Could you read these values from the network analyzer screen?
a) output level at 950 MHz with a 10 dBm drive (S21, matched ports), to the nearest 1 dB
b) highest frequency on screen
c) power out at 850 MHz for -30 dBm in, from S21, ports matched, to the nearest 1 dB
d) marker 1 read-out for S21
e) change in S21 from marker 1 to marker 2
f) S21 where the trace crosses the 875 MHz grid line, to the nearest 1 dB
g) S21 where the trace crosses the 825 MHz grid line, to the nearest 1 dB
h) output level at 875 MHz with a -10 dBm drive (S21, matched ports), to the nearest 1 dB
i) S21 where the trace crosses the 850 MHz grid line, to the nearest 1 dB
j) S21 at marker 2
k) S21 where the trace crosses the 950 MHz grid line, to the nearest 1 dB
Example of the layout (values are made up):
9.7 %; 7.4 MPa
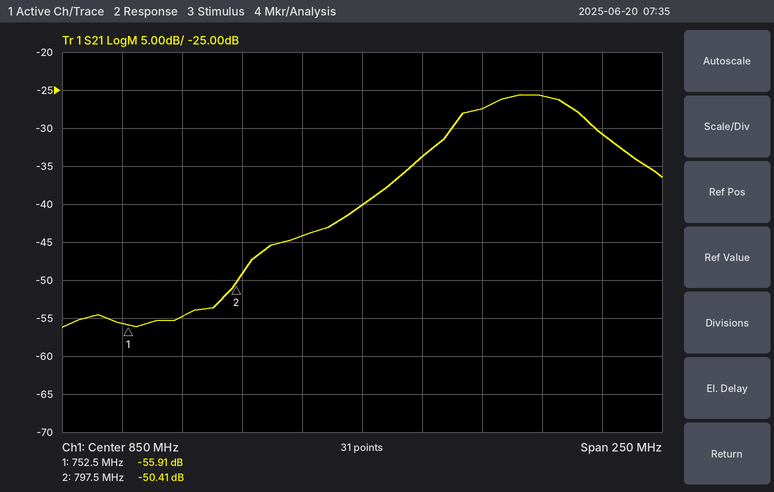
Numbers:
-21 dBm; 975 MHz; -70 dBm; -55.91 dB; 5.50 dB; -34 dB; -44 dB; -44 dBm; -40 dB; -50.41 dB; -31 dB
